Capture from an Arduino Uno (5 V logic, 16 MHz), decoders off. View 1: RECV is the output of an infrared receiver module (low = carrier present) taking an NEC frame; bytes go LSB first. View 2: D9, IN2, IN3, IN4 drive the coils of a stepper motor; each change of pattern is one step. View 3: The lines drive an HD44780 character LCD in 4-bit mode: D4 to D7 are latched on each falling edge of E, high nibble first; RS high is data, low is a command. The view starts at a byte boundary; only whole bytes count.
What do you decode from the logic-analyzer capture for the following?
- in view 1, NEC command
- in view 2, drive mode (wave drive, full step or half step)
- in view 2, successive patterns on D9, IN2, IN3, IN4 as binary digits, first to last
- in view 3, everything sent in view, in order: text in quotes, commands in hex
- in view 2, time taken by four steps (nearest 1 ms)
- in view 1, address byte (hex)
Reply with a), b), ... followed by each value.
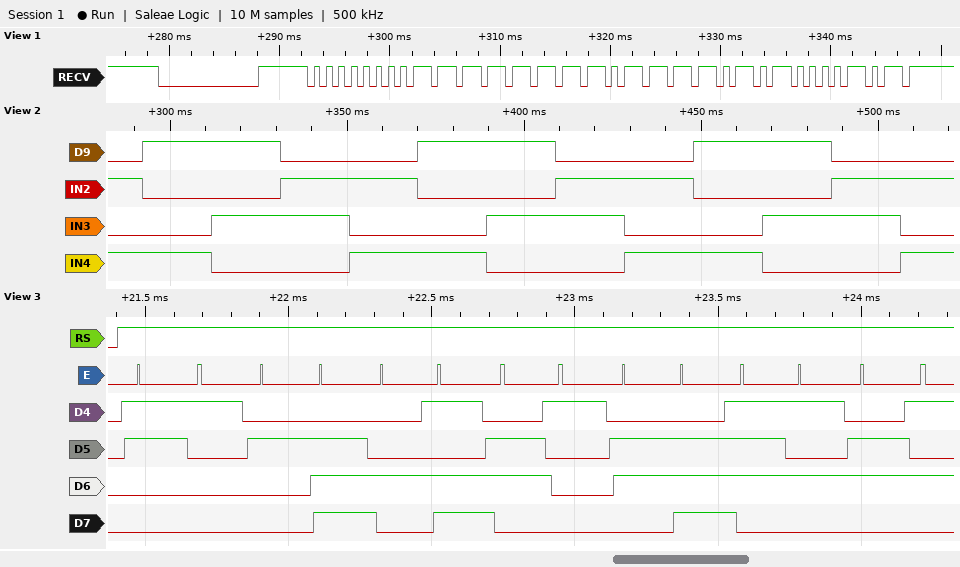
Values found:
a) 0x5E
b) full step
c) 0101 1001 1010 0110 0101 1001 1010 0110 0101 1001 1010 0110 0101
d) "1.Manue"
e) 78 ms
f) 0x00
